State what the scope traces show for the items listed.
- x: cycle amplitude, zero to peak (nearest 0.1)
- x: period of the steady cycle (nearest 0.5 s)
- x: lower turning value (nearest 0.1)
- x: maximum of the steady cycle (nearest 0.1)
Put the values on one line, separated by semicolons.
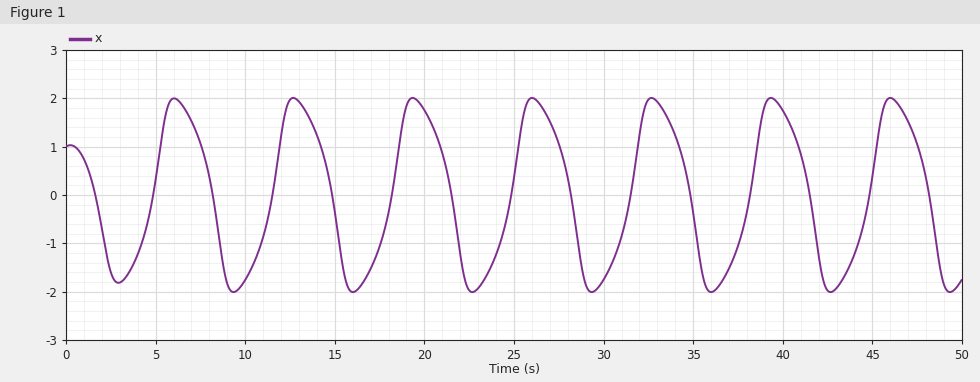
2.0; 6.5 s; -2.0; 2.0
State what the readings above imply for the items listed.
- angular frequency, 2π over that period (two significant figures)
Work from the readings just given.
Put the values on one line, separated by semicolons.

0.97 rad/s
